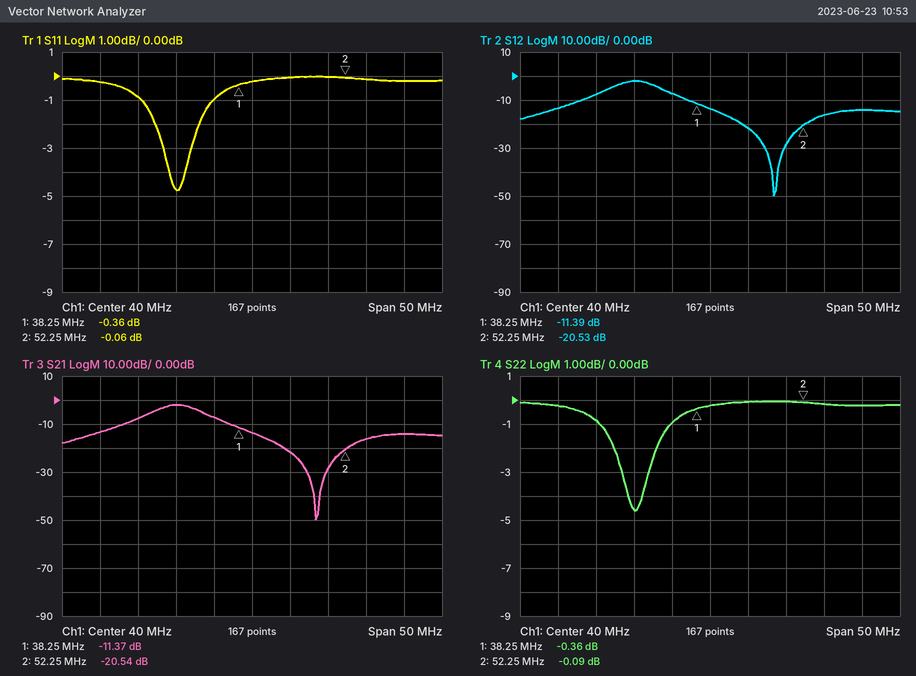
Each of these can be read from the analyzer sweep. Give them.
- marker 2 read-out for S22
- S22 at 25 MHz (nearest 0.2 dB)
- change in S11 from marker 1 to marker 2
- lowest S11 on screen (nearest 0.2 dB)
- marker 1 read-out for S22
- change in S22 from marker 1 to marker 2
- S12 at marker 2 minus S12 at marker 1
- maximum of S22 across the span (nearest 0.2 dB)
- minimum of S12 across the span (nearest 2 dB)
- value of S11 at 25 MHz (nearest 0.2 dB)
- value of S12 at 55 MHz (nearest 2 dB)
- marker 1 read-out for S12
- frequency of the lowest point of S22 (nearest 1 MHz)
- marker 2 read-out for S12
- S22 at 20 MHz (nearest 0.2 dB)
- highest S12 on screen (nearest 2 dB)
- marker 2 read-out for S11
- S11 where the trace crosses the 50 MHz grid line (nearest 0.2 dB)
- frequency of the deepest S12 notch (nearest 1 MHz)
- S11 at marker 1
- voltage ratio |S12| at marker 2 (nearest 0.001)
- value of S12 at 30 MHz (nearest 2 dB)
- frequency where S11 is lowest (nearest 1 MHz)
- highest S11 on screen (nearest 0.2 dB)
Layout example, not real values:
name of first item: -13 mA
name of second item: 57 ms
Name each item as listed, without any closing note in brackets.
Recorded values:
marker 2 read-out for S22: -0.09 dB
S22 at 25 MHz: -0.8 dB
change in S11 from marker 1 to marker 2: 0.30 dB
lowest S11 on screen: -4.8 dB
marker 1 read-out for S22: -0.36 dB
change in S22 from marker 1 to marker 2: 0.27 dB
S12 at marker 2 minus S12 at marker 1: -9.14 dB
maximum of S22 across the span: 0.0 dB
minimum of S12 across the span: -50 dB
value of S11 at 25 MHz: -0.8 dB
value of S12 at 55 MHz: -16 dB
marker 1 read-out for S12: -11.39 dB
frequency of the lowest point of S22: 30 MHz
marker 2 read-out for S12: -20.53 dB
S22 at 20 MHz: -0.2 dB
highest S12 on screen: -2 dB
marker 2 read-out for S11: -0.06 dB
S11 where the trace crosses the 50 MHz grid line: 0.0 dB
frequency of the deepest S12 notch: 48 MHz
S11 at marker 1: -0.36 dB
voltage ratio |S12| at marker 2: 0.094
value of S12 at 30 MHz: -2 dB
frequency where S11 is lowest: 30 MHz
highest S11 on screen: 0.0 dB
